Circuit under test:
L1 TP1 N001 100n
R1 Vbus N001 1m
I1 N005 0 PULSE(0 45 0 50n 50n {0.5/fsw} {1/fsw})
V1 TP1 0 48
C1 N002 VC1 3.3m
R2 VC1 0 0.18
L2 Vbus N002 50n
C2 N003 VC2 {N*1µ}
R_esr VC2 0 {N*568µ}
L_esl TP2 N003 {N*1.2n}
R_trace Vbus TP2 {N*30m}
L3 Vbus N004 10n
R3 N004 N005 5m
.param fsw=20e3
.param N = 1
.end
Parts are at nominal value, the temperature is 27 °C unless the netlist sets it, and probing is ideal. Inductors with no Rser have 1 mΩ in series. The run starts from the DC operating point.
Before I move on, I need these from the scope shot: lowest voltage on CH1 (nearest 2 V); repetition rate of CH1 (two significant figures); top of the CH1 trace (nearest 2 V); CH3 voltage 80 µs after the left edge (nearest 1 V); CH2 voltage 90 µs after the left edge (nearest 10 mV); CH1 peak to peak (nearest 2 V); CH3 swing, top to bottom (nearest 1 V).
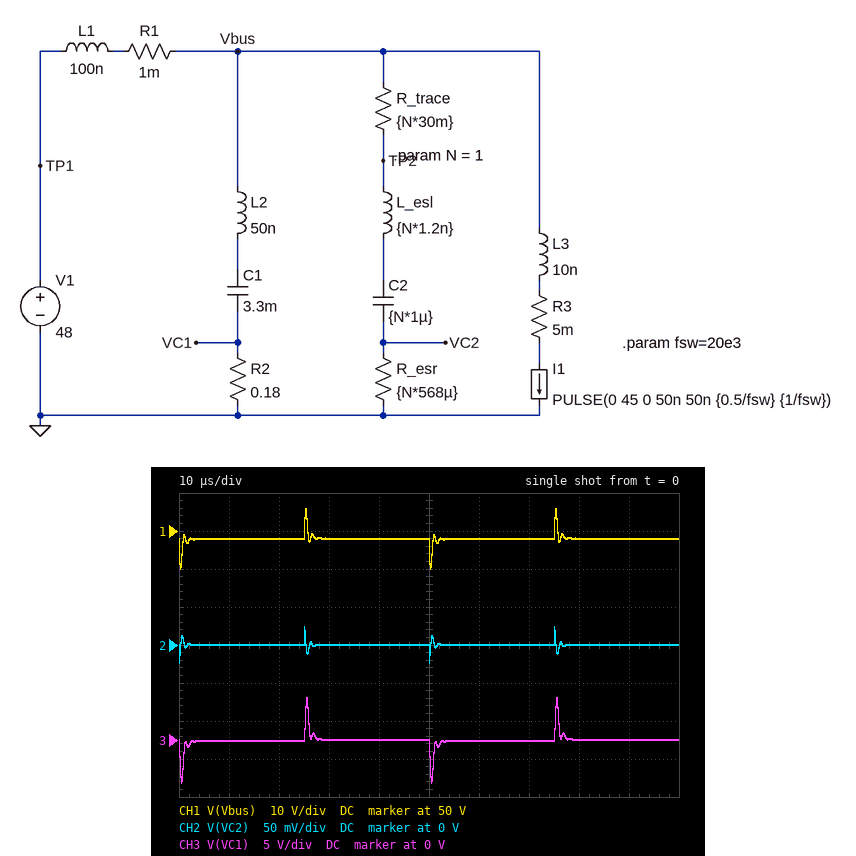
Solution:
40 V
20 kHz
56 V
0 V
0 V
16 V
11 V
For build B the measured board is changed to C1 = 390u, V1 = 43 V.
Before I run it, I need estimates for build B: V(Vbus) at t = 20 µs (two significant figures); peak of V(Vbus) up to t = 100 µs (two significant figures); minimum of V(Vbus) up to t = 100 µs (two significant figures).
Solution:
43 V
51 V
35 V
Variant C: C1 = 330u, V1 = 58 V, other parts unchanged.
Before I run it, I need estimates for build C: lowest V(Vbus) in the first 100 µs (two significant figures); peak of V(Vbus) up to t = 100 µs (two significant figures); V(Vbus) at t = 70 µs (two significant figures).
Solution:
50 V
66 V
58 V
